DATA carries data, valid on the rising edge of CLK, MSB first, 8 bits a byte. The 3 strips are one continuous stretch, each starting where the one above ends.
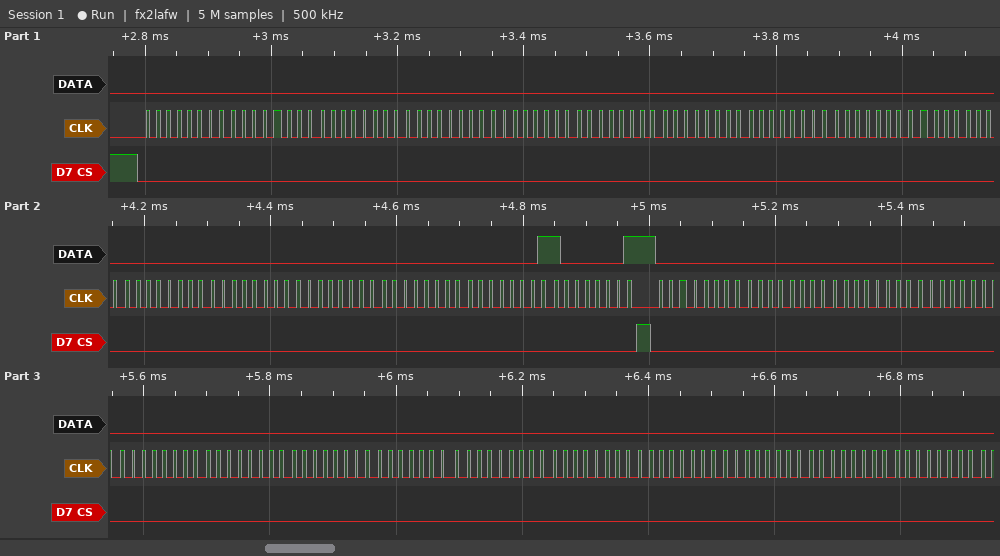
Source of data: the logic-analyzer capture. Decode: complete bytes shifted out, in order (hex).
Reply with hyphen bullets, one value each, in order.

- 00 00 00 00 00 00 00 00 00 00 00 00 00 00 01 81 00 00 00 00 00 00 00 00 00 00 00 00 00 00
